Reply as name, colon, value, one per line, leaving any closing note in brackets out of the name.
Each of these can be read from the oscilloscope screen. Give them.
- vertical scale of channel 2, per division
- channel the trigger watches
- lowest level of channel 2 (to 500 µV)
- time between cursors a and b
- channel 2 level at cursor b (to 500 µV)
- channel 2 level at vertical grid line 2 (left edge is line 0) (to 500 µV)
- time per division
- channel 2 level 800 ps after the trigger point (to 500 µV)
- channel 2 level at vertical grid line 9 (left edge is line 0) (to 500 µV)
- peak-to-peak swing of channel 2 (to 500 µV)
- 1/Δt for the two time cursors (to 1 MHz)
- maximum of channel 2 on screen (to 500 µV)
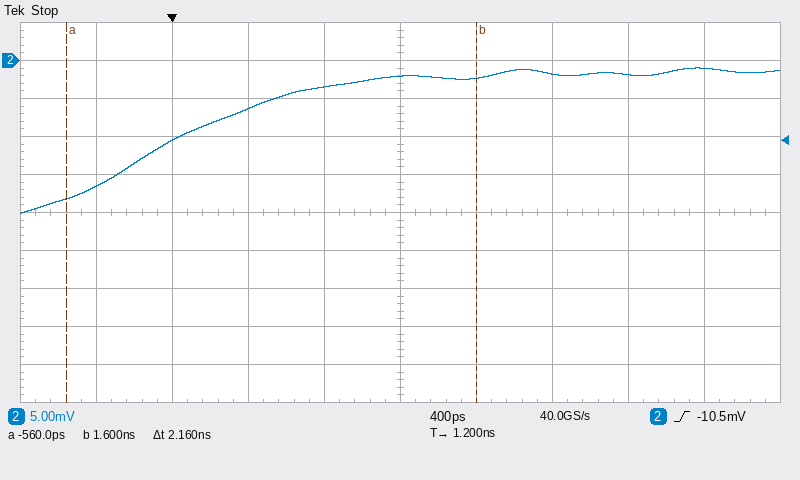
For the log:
vertical scale of channel 2, per division: 5 mV
channel the trigger watches: channel 2
lowest level of channel 2: -20.0 mV
time between cursors a and b: 2.16 ns
channel 2 level at cursor b: -2.5 mV
channel 2 level at vertical grid line 2 (left edge is line 0): -10.5 mV
time per division: 400 ps
channel 2 level 800 ps after the trigger point: -3.5 mV
channel 2 level at vertical grid line 9 (left edge is line 0): -1.0 mV
peak-to-peak swing of channel 2: 19.0 mV
1/Δt for the two time cursors: 463 MHz
maximum of channel 2 on screen: -1.0 mV
